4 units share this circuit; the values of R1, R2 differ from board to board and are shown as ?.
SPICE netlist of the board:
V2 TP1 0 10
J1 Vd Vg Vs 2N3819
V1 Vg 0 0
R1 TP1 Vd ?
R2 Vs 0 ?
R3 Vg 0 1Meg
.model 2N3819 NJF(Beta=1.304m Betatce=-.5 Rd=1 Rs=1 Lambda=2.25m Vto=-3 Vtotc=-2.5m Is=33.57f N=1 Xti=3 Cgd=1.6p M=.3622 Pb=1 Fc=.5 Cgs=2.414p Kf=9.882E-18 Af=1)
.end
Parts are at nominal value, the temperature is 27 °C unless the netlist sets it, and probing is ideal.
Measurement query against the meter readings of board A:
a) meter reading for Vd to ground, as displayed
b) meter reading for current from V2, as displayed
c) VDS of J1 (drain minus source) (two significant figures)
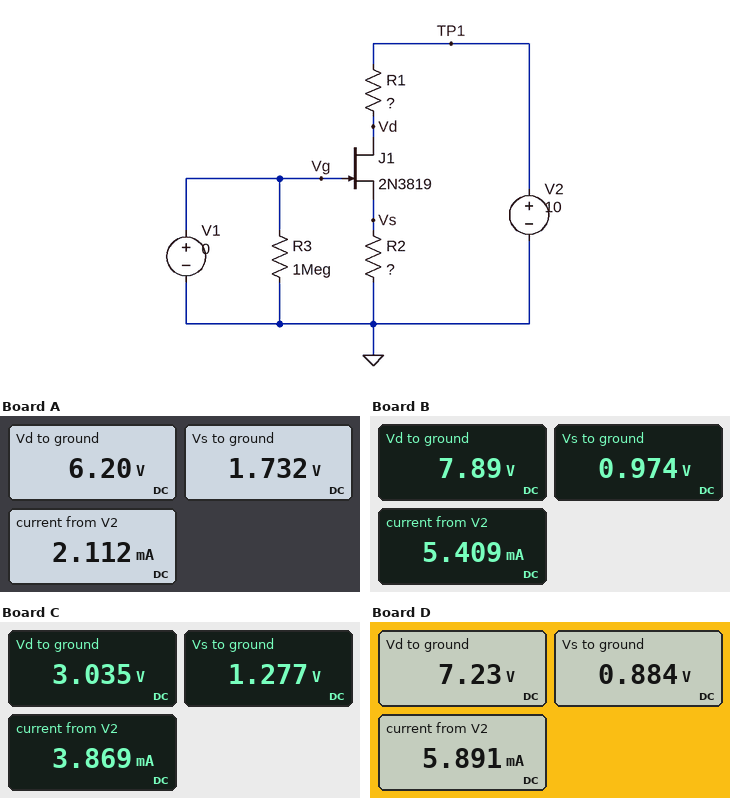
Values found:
6.20 V
2.112 mA
4.5 V
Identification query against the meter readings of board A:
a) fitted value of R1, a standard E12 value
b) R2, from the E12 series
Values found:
1.8 kΩ
820 Ω
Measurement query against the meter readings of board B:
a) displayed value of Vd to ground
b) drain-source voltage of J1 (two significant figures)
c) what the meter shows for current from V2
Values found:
7.89 V
6.9 V
5.409 mA
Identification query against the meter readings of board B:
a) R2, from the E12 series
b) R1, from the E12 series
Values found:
180 Ω
390 Ω
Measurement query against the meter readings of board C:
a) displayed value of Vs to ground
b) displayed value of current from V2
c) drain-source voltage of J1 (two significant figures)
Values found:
1.277 V
3.869 mA
1.8 V
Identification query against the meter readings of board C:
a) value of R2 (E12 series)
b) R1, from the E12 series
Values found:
330 Ω
1.8 kΩ
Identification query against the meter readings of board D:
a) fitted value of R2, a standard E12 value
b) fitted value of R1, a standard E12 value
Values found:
150 Ω
470 Ω
